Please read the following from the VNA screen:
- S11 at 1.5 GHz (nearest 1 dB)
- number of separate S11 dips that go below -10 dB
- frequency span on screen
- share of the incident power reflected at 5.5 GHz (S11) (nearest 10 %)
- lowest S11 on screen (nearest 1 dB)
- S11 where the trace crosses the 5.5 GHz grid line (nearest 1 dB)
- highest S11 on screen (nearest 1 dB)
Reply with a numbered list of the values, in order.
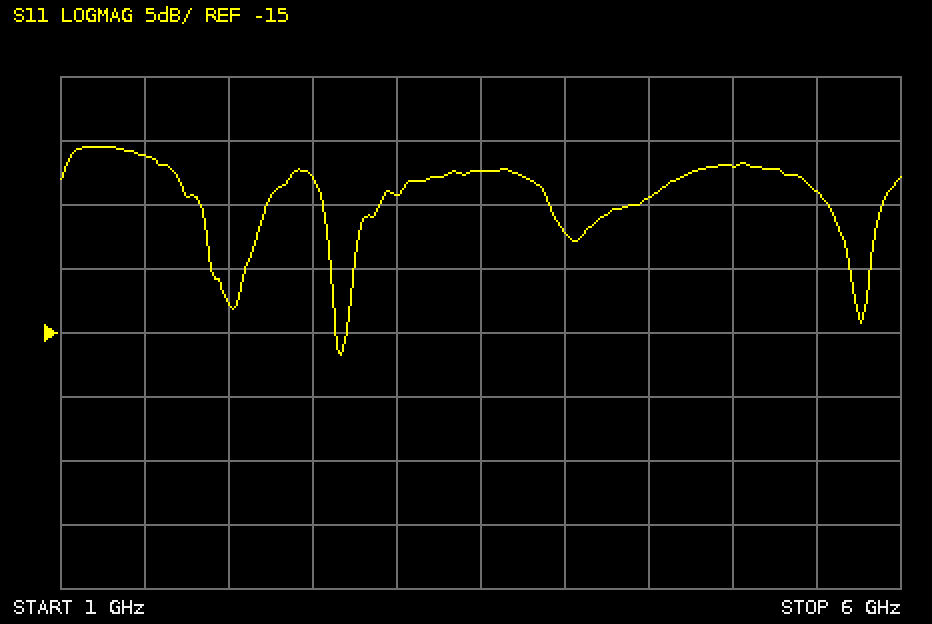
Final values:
1. -1 dB
2. 3
3. 5 GHz
4. 40 %
5. -17 dB
6. -4 dB
7. 0 dB
